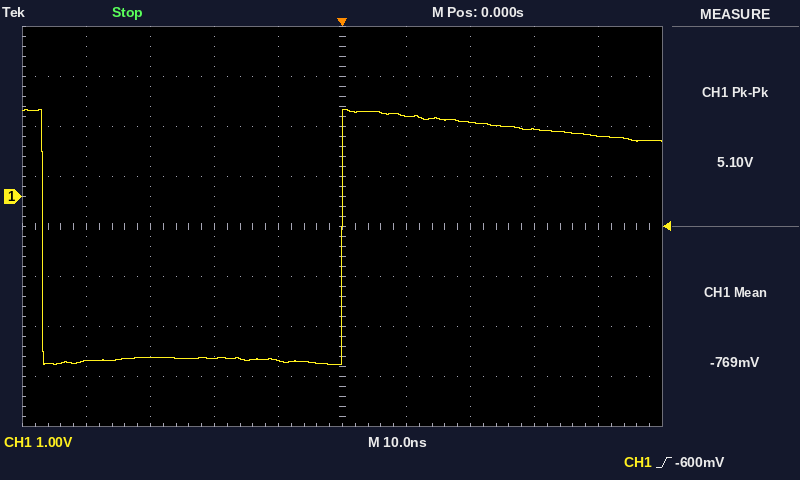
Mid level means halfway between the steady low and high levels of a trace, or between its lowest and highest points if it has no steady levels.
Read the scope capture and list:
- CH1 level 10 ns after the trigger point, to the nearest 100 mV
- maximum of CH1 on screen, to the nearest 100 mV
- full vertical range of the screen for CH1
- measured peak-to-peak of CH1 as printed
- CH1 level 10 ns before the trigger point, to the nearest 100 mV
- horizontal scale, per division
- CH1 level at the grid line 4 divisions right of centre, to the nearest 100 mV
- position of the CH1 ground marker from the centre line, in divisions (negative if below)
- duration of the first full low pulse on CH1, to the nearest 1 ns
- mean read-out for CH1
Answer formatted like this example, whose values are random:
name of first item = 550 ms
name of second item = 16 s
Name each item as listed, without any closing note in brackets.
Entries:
CH1 level 10 ns after the trigger point, to the nearest 100 mV = 1.6 V
maximum of CH1 on screen, to the nearest 100 mV = 1.7 V
full vertical range of the screen for CH1 = 8 V
measured peak-to-peak of CH1 as printed = 5.10 V
CH1 level 10 ns before the trigger point, to the nearest 100 mV = -3.3 V
horizontal scale, per division = 10 ns
CH1 level at the grid line 4 divisions right of centre, to the nearest 100 mV = 1.2 V
position of the CH1 ground marker from the centre line, in divisions = +0.6 div
duration of the first full low pulse on CH1, to the nearest 1 ns = 47 ns
mean read-out for CH1 = -769 mV
